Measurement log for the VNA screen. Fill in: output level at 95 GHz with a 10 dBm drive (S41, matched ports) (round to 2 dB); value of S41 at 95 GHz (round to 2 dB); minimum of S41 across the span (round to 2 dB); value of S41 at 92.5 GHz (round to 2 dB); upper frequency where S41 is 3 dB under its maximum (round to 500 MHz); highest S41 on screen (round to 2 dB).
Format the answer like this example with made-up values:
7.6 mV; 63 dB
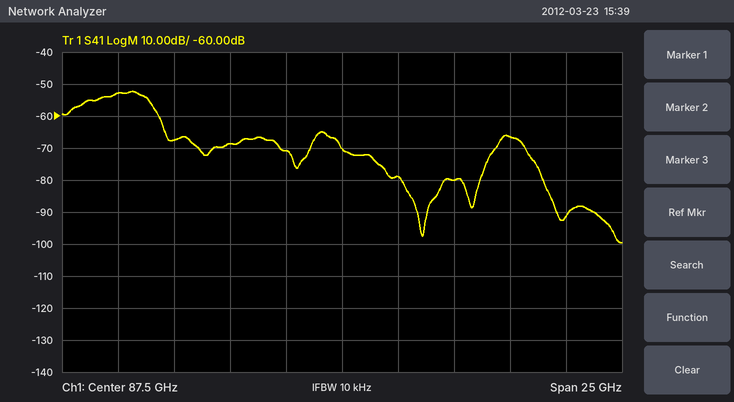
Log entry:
-56 dBm; -66 dB; -100 dB; -80 dB; 79.0 GHz; -52 dB
